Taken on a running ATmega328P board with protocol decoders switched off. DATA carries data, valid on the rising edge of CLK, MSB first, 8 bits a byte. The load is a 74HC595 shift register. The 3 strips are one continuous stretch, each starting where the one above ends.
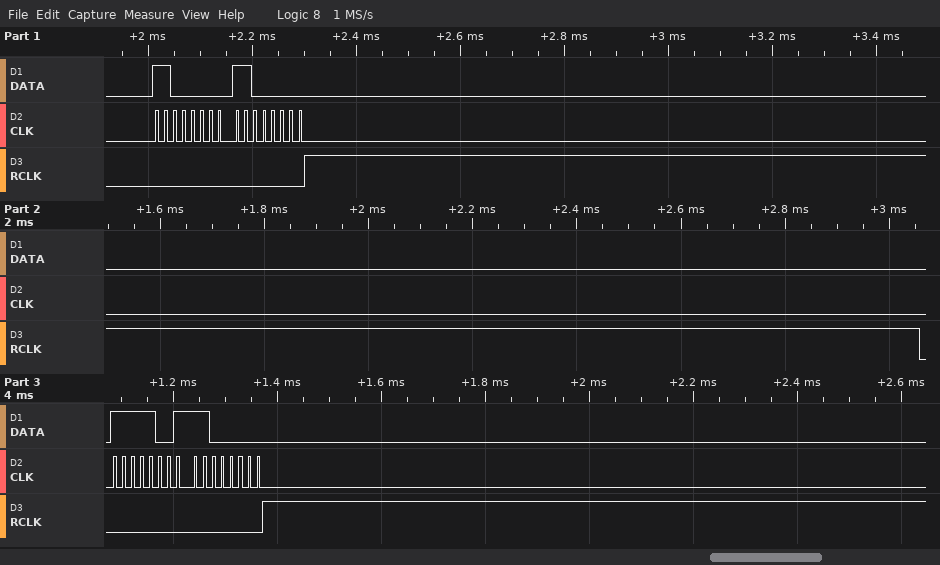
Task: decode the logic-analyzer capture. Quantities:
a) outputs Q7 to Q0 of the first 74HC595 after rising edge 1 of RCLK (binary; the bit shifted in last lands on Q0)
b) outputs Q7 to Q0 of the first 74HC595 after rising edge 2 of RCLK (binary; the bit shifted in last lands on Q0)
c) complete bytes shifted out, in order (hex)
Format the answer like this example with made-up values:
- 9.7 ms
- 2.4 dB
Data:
- 11000000
- 11000000
- C0 C0 F9 C0
